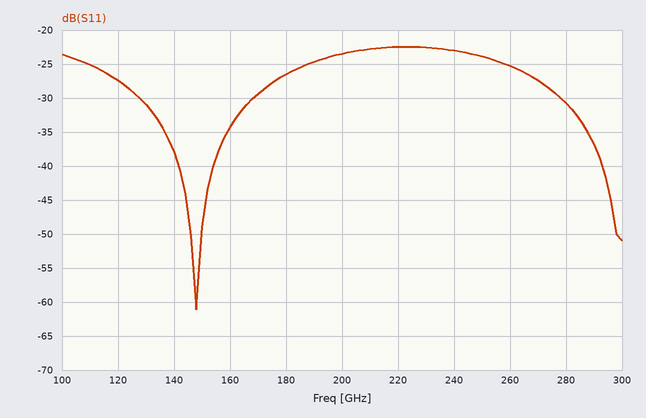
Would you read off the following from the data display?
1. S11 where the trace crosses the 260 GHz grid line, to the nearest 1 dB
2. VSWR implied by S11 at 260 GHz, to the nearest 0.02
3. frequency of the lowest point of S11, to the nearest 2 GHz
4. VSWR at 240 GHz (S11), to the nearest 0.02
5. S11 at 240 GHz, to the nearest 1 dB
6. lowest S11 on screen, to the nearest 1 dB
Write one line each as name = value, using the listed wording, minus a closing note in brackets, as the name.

S11 where the trace crosses the 260 GHz grid line, to the nearest 1 dB = -25 dB
VSWR implied by S11 at 260 GHz, to the nearest 0.02 = 1.12
frequency of the lowest point of S11, to the nearest 2 GHz = 148 GHz
VSWR at 240 GHz (S11), to the nearest 0.02 = 1.16
S11 at 240 GHz, to the nearest 1 dB = -23 dB
lowest S11 on screen, to the nearest 1 dB = -61 dB
